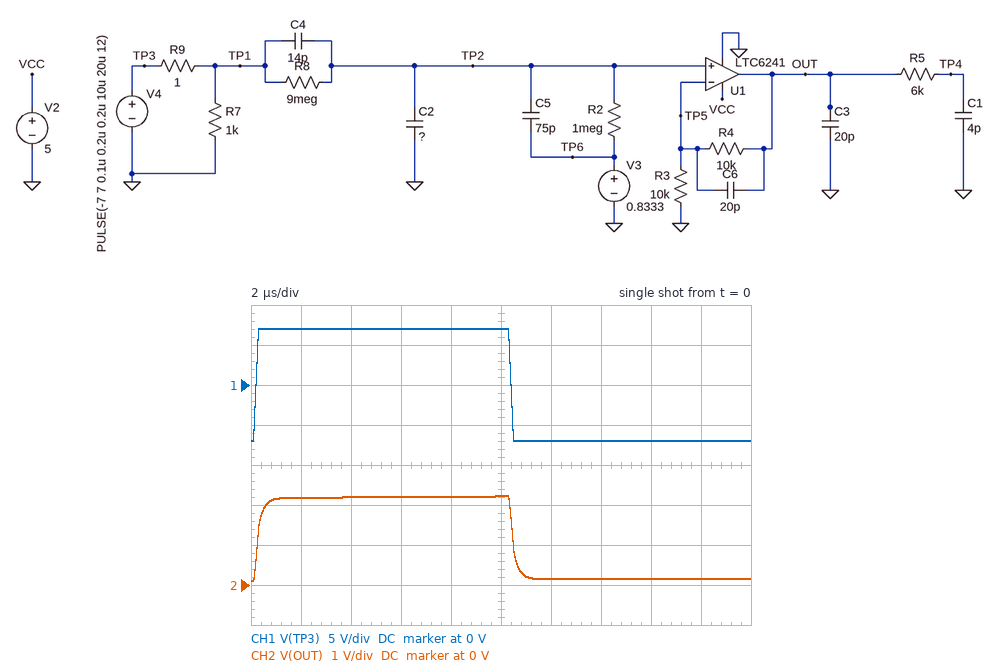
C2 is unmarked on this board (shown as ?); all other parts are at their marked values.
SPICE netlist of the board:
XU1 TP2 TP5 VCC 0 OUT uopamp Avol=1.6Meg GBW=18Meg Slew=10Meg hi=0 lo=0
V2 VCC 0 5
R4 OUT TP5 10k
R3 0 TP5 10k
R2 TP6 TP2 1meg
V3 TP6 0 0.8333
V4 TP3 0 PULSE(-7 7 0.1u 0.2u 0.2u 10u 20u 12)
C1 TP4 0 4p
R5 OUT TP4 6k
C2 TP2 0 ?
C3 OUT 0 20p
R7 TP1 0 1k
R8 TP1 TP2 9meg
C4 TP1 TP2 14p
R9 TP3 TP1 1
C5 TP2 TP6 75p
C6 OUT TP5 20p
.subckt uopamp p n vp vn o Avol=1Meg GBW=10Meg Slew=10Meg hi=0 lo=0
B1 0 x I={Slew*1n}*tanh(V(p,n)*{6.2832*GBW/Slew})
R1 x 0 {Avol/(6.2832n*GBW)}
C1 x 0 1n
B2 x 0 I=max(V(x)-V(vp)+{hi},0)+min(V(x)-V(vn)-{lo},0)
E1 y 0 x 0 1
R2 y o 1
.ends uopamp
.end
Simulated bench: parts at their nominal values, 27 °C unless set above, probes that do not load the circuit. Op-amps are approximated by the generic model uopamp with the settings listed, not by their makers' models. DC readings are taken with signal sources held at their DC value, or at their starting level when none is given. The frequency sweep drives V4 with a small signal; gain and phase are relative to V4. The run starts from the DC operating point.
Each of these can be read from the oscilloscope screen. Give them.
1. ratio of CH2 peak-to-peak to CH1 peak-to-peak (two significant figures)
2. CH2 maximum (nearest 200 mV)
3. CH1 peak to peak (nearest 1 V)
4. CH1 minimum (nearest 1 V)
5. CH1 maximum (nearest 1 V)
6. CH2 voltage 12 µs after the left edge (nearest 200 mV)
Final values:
0.15
2.2 V
14 V
-7 V
7 V
200 mV
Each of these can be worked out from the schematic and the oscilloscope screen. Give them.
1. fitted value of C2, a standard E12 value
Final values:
100 pF
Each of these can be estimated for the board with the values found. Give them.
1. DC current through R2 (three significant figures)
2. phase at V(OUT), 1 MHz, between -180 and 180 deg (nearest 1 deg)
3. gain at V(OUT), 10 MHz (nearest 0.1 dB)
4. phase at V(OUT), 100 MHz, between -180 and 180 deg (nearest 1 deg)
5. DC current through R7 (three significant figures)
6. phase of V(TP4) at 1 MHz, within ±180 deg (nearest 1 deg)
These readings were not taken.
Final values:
783 nA
-24 deg
-24.0 dB
-81 deg
6.99 mA
-32 deg
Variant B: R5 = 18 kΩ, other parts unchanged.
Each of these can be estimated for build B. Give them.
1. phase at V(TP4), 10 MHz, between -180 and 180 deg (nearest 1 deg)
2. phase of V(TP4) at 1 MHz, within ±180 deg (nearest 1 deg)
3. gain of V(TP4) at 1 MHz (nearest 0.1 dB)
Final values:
-110 deg
-48 deg
-20.3 dB
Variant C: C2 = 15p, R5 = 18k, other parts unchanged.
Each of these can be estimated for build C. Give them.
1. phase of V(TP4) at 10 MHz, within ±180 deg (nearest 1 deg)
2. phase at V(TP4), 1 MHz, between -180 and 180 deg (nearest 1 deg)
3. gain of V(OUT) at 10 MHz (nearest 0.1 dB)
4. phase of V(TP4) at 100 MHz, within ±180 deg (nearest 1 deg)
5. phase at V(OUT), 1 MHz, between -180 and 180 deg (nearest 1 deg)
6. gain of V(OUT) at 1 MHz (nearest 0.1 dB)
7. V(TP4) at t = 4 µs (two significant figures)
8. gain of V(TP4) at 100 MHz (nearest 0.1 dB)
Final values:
-110 deg
-48 deg
-18.8 dB
-170 deg
-24 deg
-14.3 dB
3.8 V
-65.6 dB
